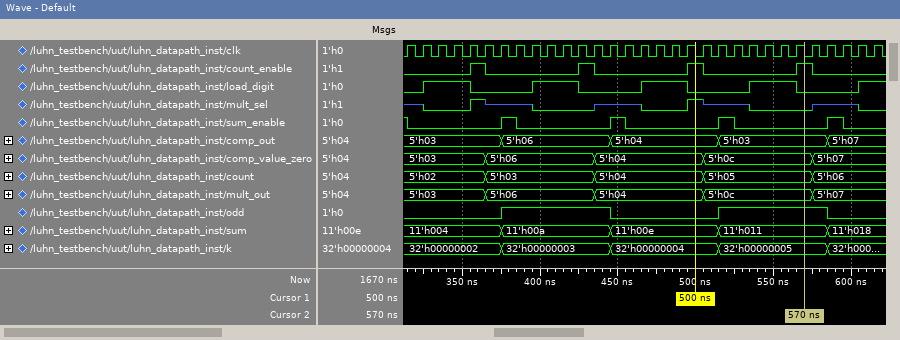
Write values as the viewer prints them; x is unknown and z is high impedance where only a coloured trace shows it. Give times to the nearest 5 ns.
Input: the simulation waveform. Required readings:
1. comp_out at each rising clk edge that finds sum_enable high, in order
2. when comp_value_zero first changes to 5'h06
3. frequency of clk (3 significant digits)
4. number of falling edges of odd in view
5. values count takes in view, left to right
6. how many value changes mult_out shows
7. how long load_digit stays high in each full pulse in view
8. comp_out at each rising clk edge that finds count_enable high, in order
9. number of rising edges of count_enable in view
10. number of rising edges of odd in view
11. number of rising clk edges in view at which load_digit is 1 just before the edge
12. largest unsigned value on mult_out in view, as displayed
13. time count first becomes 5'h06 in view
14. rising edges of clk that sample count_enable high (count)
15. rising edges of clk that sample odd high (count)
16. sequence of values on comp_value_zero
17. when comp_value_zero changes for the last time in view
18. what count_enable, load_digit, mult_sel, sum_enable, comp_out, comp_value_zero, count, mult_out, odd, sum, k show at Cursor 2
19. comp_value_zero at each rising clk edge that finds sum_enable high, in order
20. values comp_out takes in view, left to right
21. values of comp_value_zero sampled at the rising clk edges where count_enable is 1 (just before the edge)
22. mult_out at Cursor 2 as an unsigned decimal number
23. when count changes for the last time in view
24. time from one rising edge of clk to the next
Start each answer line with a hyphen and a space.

- 5'h03, 5'h06, 5'h04, 5'h03, 5'h07
- 365 ns
- 100 MHz
- 2
- 5'h02, 5'h03, 5'h04, 5'h05, 5'h06
- 4
- 30 ns, 30 ns, 30 ns, 30 ns
- 5'h03, 5'h06, 5'h04, 5'h03
- 4
- 2
- 13
- 5'h0c
- 575 ns
- 4
- 14
- 5'h03, 5'h06, 5'h04, 5'h0c, 5'h07
- 575 ns
- count_enable=1, load_digit=0, mult_sel=0, sum_enable=0, comp_out=5'h03, comp_value_zero=5'h0c, count=5'h05, mult_out=5'h0c, odd=1, sum=11'h011, k=32'h00000005
- 5'h03, 5'h06, 5'h04, 5'h0c, 5'h07
- 5'h03, 5'h06, 5'h04, 5'h03, 5'h07
- 5'h03, 5'h06, 5'h04, 5'h0c
- 12
- 575 ns
- 10 ns
